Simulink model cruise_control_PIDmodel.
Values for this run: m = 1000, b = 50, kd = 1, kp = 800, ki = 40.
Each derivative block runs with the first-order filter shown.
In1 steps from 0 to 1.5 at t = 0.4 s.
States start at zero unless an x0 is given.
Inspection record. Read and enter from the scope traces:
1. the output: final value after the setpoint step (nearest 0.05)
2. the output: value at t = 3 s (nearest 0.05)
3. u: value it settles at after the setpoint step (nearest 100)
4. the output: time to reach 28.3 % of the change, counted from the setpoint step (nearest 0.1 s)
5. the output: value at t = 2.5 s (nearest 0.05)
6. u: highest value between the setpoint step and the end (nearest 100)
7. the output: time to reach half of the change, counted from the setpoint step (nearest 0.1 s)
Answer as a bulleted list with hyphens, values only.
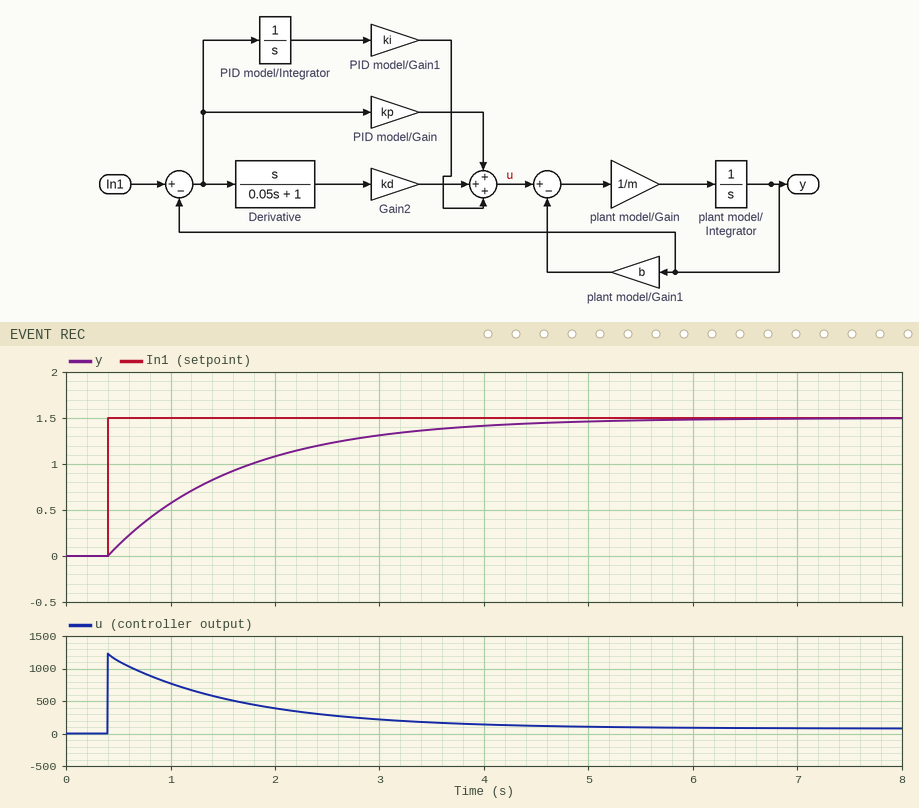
- 1.50
- 1.30
- 100
- 0.4 s
- 1.20
- 1200
- 0.9 s
